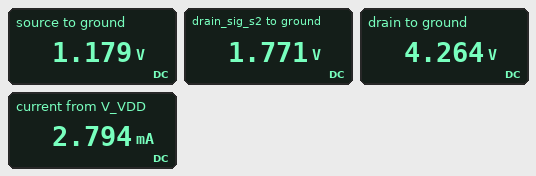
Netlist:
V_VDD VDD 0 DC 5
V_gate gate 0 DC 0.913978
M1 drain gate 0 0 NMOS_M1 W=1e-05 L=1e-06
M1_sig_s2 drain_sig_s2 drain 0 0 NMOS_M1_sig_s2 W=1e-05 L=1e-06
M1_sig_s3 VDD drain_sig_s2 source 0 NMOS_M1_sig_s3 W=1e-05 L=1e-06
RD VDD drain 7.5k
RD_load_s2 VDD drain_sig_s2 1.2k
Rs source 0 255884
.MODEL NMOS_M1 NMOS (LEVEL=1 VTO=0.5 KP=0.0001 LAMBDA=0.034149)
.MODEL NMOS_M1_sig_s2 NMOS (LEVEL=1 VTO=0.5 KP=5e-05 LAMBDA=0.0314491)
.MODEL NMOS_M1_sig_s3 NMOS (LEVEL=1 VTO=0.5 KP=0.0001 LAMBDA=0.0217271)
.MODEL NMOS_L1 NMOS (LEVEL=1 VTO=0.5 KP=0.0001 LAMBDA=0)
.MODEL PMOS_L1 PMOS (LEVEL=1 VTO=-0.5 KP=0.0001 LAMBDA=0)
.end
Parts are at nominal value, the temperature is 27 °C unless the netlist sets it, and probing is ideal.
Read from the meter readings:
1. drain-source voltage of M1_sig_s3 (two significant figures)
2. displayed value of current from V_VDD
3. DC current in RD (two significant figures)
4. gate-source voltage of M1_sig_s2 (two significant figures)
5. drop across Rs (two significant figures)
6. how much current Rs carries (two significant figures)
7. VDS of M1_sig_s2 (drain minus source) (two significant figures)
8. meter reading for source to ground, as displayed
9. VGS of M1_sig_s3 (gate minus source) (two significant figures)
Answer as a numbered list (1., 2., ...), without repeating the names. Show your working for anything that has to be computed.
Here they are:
1. 5 V - 1.179 V = 3.8 V
2. 2.794 mA
3. (5 V - 4.264 V) / 7.5 kΩ = 98 µA
4. 4.264 V = 4.3 V
5. 1.179 V = 1.2 V
6. (1.179 V) / 255.9 kΩ = 4.6 µA
7. 1.771 V = 1.8 V
8. 1.179 V
9. 1.771 V - 1.179 V = 590 mV
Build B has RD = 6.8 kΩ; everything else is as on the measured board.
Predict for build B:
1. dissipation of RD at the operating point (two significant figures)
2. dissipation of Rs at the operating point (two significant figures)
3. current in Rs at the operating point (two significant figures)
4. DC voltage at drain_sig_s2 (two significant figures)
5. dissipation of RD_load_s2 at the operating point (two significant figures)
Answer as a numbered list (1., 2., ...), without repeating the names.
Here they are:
1. 66 µW
2. 5.2 µW
3. 4.5 µA
4. 1.7 V
5. 8.9 mW
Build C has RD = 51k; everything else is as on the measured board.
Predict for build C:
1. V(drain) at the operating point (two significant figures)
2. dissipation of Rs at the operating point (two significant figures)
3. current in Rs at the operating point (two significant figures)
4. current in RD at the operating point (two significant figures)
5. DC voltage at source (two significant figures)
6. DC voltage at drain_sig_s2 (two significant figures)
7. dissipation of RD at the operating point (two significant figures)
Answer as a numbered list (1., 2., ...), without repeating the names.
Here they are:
1. 550 mV
2. 73 µW
3. 17 µA
4. 87 µA
5. 4.3 V
6. 5.0 V
7. 390 µW
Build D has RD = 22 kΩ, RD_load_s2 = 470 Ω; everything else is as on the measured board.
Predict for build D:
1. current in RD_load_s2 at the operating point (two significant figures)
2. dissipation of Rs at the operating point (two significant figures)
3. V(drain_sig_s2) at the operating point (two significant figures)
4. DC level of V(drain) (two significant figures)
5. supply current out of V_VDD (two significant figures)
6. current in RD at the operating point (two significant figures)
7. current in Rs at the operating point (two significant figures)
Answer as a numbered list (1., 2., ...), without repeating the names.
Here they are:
1. 1.7 mA
2. 49 µW
3. 4.2 V
4. 2.9 V
5. 1.8 mA
6. 94 µA
7. 14 µA
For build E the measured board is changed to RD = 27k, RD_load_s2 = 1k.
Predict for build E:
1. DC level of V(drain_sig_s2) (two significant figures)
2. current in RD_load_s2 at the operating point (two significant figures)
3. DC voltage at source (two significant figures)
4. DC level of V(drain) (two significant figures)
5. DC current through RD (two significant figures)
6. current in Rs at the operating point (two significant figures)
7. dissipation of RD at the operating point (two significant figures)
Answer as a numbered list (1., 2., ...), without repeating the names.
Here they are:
1. 3.9 V
2. 1.1 mA
3. 3.2 V
4. 2.5 V
5. 93 µA
6. 13 µA
7. 230 µW
